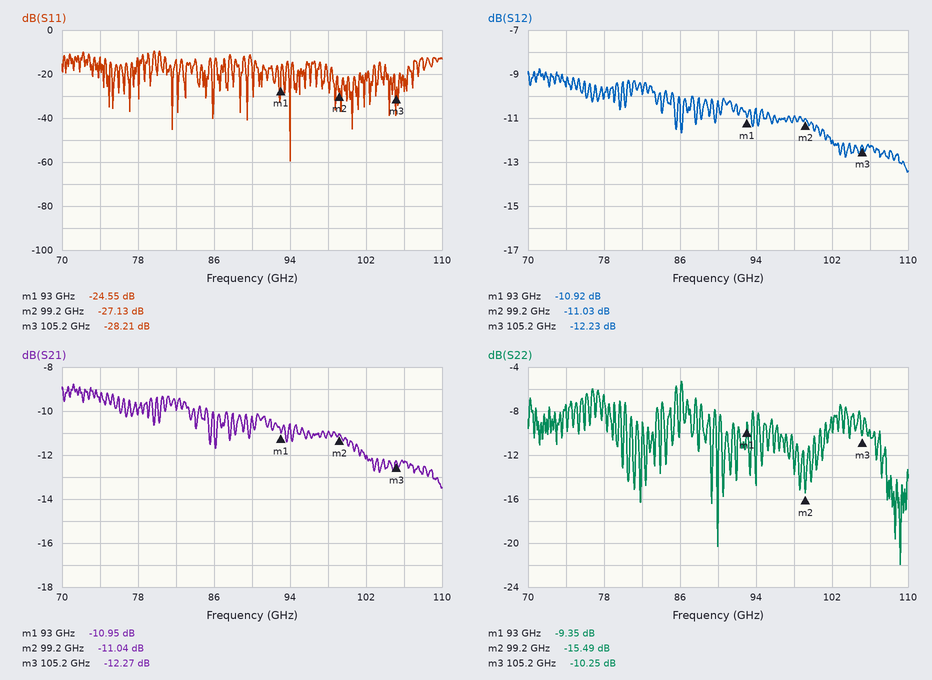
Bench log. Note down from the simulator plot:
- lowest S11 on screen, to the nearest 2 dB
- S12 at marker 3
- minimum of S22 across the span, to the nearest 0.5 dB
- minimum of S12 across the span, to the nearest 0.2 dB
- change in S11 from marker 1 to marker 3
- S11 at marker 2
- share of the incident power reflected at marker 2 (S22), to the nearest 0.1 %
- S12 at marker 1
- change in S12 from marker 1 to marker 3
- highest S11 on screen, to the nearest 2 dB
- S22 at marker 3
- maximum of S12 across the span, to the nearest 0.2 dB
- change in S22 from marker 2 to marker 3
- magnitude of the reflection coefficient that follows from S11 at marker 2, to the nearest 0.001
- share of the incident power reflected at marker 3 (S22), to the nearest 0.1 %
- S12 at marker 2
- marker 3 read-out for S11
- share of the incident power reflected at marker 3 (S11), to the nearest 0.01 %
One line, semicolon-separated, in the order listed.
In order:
-60 dB; -12.23 dB; -22.0 dB; -13.4 dB; -3.66 dB; -27.13 dB; 2.8 %; -10.92 dB; -1.31 dB; -10 dB; -10.25 dB; -8.8 dB; 5.24 dB; 0.044; 9.4 %; -11.03 dB; -28.21 dB; 0.15 %
